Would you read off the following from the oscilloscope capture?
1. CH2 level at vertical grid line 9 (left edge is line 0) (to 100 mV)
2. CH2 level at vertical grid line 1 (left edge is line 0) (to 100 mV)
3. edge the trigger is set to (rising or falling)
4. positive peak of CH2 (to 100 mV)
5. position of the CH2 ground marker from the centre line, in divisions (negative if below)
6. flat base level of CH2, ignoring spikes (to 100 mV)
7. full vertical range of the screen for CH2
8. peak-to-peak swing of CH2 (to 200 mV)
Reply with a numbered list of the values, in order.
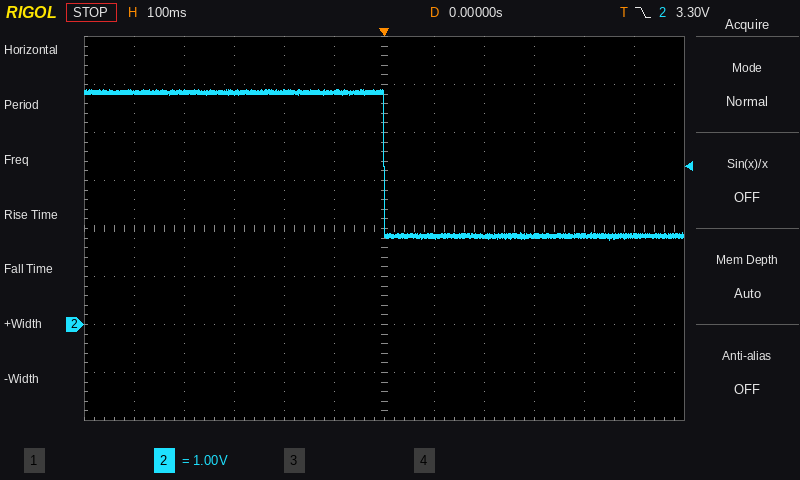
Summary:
1. 1.8 V
2. 4.8 V
3. falling
4. 4.9 V
5. -2.0 div
6. 1.8 V
7. 8 V
8. 3.2 V
